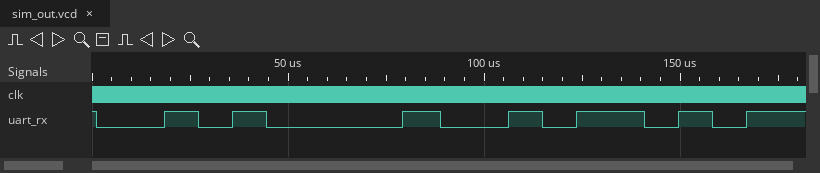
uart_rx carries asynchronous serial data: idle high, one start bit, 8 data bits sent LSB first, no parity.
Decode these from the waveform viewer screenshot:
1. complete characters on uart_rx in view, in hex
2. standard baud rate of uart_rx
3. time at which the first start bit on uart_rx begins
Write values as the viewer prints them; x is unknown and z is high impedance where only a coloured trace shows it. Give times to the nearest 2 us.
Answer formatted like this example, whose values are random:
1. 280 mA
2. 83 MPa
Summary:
1. 0A, 5A
2. 115200 baud
3. 0 us
